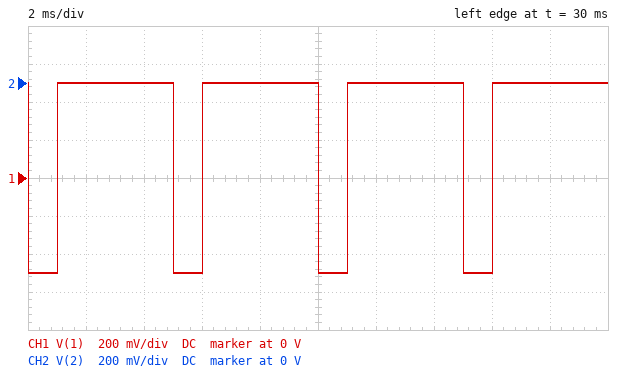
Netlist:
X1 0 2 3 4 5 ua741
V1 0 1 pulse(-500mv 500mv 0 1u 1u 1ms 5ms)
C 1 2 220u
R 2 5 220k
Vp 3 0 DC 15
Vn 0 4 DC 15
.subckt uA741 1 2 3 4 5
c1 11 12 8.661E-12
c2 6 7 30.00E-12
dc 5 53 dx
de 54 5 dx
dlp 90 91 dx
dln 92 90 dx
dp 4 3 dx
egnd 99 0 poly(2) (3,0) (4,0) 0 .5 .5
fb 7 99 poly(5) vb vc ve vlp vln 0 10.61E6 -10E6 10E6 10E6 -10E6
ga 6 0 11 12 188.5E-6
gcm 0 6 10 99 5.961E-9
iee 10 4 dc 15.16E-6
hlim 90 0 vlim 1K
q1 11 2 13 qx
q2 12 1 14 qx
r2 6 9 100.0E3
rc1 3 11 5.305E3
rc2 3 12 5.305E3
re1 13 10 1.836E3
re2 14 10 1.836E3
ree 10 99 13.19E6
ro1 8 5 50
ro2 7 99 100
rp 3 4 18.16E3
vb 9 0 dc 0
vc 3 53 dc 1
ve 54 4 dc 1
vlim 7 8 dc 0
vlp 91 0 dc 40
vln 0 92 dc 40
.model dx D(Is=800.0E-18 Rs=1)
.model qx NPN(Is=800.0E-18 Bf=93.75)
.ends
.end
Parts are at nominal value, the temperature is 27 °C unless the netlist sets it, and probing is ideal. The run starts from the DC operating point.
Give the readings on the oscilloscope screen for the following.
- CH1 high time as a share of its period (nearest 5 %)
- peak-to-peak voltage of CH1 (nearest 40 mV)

80 %
1.00 V
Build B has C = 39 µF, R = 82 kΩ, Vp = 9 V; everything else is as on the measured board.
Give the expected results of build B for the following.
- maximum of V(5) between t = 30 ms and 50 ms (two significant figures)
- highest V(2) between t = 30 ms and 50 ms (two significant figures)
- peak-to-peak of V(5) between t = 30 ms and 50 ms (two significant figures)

8.6 V
3.3 mV
23 V
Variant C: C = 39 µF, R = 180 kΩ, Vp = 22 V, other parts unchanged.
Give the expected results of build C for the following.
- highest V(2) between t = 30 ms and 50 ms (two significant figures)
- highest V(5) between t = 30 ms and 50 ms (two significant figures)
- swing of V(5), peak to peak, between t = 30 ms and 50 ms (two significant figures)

3.8 mV
22 V
36 V
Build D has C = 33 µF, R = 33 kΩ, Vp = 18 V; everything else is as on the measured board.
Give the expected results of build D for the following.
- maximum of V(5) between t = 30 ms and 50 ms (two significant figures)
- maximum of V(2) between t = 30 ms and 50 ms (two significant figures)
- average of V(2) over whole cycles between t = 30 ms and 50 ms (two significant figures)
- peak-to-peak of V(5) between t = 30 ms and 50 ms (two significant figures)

18 V
23 mV
-190 mV
32 V
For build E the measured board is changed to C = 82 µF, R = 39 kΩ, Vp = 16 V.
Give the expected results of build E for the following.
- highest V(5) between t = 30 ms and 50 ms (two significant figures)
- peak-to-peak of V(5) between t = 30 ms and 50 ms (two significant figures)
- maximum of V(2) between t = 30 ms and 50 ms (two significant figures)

16 V
30 V
5.7 mV
